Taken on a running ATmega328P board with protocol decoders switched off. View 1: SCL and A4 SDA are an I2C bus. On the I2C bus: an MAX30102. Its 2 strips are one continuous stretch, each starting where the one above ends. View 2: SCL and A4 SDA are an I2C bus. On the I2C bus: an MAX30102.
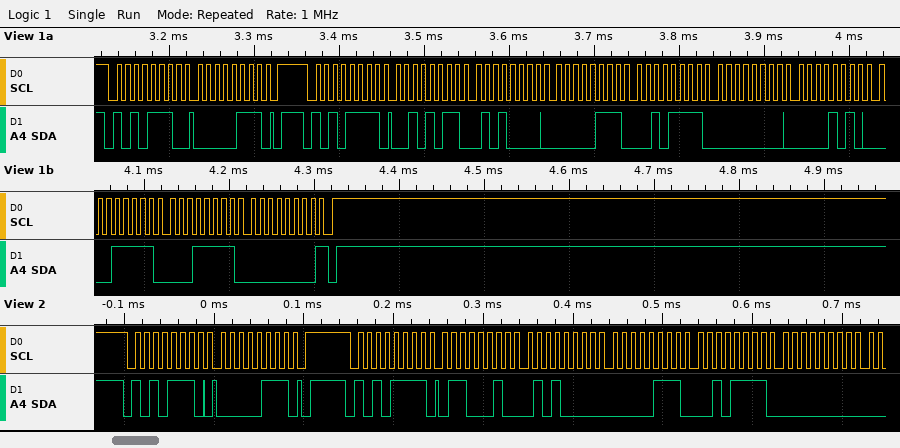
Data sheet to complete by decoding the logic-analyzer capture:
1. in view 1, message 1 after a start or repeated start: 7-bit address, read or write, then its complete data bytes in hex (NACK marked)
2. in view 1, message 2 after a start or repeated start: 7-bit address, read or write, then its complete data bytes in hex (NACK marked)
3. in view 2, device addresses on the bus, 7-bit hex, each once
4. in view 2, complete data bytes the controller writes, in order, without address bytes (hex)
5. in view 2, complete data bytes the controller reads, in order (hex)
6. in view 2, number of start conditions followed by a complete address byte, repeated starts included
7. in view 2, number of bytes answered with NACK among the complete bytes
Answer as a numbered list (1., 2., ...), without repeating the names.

1. 0x57 write: 07
2. 0x57 read: 2B 50 07 2F 00 0A 1F 1F 00 NACK
3. 0x57
4. 07
5. 62 50 07 2F 00
6. 2
7. 0
